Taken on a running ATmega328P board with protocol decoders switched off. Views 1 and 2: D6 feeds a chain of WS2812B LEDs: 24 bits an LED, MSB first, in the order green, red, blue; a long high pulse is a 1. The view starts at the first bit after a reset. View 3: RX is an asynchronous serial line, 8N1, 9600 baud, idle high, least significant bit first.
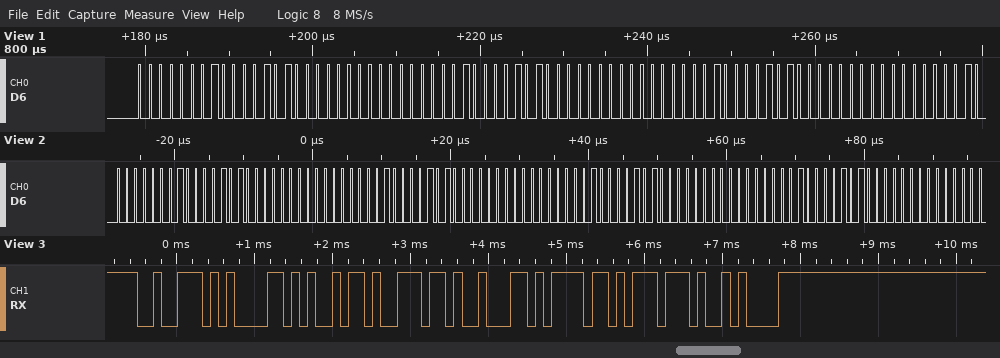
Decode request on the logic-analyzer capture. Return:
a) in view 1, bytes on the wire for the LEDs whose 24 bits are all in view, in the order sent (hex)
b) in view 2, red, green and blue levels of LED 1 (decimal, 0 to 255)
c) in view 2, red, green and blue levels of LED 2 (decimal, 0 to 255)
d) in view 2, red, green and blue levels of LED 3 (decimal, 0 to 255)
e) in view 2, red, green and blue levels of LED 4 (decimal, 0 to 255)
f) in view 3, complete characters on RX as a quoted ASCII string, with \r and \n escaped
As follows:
01 0A 00 01 0A 00 01 0A 00
10, 1, 0
10, 1, 0
10, 1, 0
10, 1, 0
"rainbow\n"
